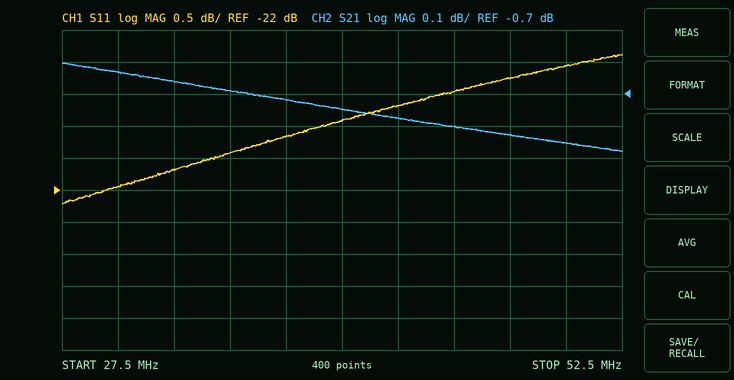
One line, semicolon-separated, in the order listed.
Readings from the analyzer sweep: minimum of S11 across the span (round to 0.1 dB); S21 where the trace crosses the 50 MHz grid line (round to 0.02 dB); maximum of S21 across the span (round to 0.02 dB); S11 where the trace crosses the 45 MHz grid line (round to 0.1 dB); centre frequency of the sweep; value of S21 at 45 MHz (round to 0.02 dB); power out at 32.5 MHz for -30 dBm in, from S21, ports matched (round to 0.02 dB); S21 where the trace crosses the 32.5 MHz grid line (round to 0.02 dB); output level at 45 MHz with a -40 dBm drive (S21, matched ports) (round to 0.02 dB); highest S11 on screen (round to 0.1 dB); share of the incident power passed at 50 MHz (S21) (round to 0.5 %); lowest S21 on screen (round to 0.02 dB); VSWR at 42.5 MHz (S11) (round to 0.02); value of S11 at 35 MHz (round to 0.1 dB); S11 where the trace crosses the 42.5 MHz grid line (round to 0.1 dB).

-22.2 dB; -0.86 dB; -0.60 dB; -20.5 dB; 40 MHz; -0.80 dB; -30.66 dBm; -0.66 dB; -40.80 dBm; -19.9 dB; 82.0 %; -0.88 dB; 1.20; -21.4 dB; -20.7 dB
